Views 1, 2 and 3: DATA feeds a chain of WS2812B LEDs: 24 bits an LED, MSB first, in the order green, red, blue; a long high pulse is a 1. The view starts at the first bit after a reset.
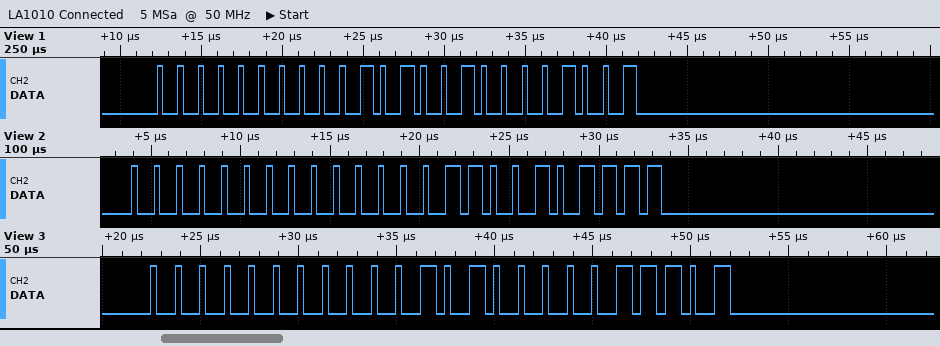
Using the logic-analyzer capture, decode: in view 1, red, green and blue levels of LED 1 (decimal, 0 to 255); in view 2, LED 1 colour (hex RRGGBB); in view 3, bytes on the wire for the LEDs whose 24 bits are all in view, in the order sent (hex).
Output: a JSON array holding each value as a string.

["41, 0, 9", "#03002F", "00 14 1D"]
